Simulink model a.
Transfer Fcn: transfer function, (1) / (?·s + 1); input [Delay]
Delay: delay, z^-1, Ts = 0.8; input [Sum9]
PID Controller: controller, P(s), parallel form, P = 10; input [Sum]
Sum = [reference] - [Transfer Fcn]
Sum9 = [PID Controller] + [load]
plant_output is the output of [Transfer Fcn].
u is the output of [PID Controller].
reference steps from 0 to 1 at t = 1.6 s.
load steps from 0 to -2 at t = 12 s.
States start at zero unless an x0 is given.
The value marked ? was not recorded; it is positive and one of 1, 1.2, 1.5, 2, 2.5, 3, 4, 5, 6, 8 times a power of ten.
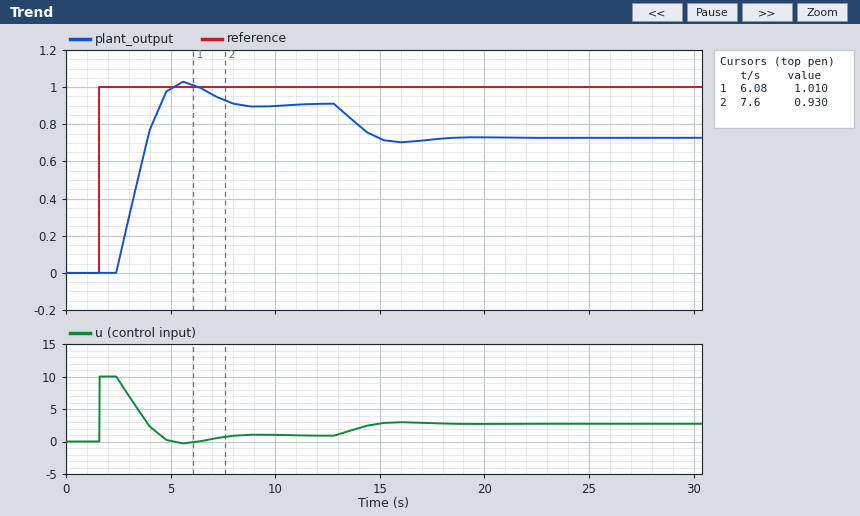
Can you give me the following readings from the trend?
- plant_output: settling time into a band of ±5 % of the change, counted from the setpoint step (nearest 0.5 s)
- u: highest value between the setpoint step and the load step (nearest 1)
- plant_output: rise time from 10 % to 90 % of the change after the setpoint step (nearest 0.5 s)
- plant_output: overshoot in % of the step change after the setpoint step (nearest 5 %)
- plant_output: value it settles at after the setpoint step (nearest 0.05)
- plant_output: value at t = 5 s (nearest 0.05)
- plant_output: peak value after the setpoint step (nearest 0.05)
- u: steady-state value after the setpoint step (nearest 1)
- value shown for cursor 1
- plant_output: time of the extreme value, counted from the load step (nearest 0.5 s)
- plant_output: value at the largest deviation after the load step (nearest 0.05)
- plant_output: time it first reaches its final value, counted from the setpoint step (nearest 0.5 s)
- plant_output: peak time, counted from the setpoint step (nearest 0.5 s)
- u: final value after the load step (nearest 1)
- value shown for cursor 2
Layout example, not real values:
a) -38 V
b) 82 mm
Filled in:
a) 5.5 s
b) 10
c) 1.5 s
d) 15 %
e) 0.90
f) 1.00
g) 1.05
h) 1
i) 1.010
j) 4.0 s
k) 0.70
l) 3.0 s
m) 4.0 s
n) 3
o) 0.930
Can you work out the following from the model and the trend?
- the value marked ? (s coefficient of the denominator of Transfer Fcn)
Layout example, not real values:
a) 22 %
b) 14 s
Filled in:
a) 20
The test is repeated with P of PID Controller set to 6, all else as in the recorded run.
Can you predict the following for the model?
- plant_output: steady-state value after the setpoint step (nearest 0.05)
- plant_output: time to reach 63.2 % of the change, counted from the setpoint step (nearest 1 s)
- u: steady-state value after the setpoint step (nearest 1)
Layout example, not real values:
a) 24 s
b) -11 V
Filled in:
a) 0.85
b) 3 s
c) 1
